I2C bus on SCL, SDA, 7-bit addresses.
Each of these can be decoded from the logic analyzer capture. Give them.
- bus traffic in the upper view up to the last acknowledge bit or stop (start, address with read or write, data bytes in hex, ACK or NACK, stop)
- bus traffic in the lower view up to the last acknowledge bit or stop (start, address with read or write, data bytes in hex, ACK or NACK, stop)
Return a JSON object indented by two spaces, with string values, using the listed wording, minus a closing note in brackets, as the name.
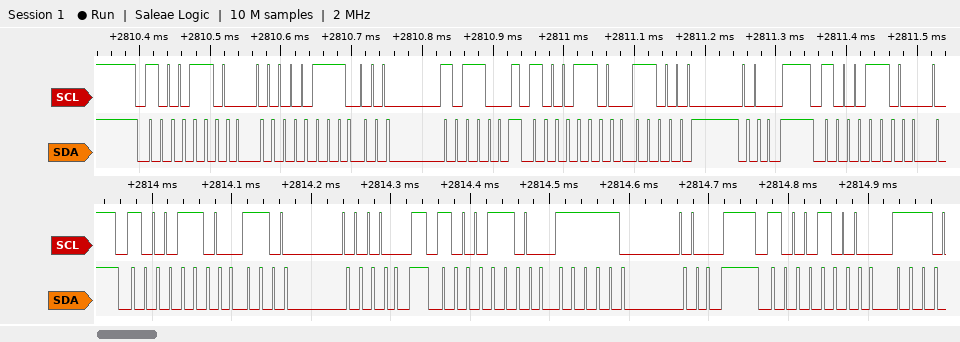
{
  "bus traffic in the upper view up to the last acknowledge bit or stop": "start, address 46 write ACK, 07 ACK, 16 ACK, stop, start, address 46 write ACK, C0 ACK, stop, start, address 46 write ACK",
  "bus traffic in the lower view up to the last acknowledge bit or stop": "start, address 46 write ACK, C0 ACK, stop, start, address 46 write ACK, F8 ACK, stop, start, address 44 write ACK"
}
